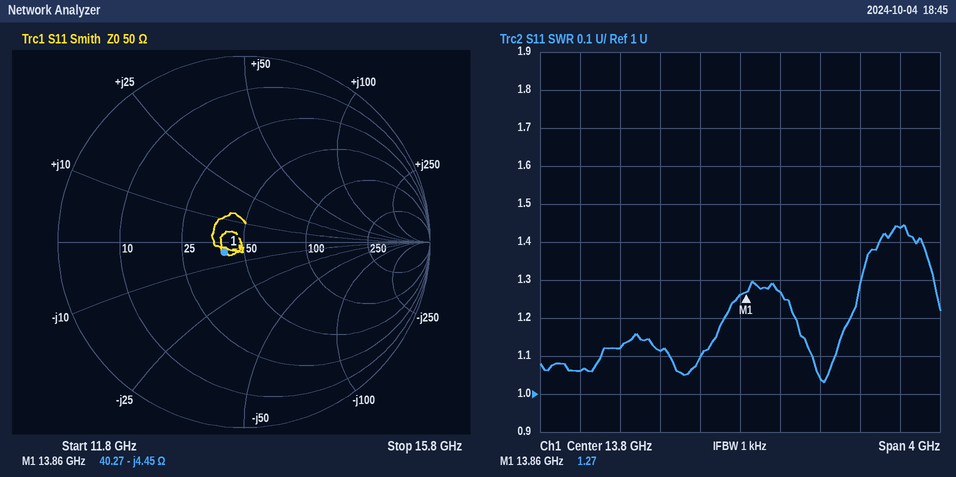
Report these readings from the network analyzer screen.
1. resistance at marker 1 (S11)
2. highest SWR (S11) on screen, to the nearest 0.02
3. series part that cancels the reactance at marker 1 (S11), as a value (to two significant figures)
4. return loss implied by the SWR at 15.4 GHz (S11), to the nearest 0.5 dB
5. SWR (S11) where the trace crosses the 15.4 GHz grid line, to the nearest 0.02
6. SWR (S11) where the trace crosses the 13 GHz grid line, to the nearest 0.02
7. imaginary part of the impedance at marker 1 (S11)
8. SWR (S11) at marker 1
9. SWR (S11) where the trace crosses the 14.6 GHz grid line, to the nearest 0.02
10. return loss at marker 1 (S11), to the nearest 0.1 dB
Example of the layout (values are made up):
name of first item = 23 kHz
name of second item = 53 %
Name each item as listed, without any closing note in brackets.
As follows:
resistance at marker 1 = 40.27 Ω
highest SWR (S11) on screen, to the nearest 0.02 = 1.44
series part that cancels the reactance at marker 1 (S11), as a value = 51 pH
return loss implied by the SWR at 15.4 GHz (S11), to the nearest 0.5 dB = 15.0 dB
SWR (S11) where the trace crosses the 15.4 GHz grid line, to the nearest 0.02 = 1.44
SWR (S11) where the trace crosses the 13 GHz grid line, to the nearest 0.02 = 1.12
imaginary part of the impedance at marker 1 = -4.45 Ω
SWR (S11) at marker 1 = 1.27
SWR (S11) where the trace crosses the 14.6 GHz grid line, to the nearest 0.02 = 1.04
return loss at marker 1 (S11), to the nearest 0.1 dB = 18.5 dB
